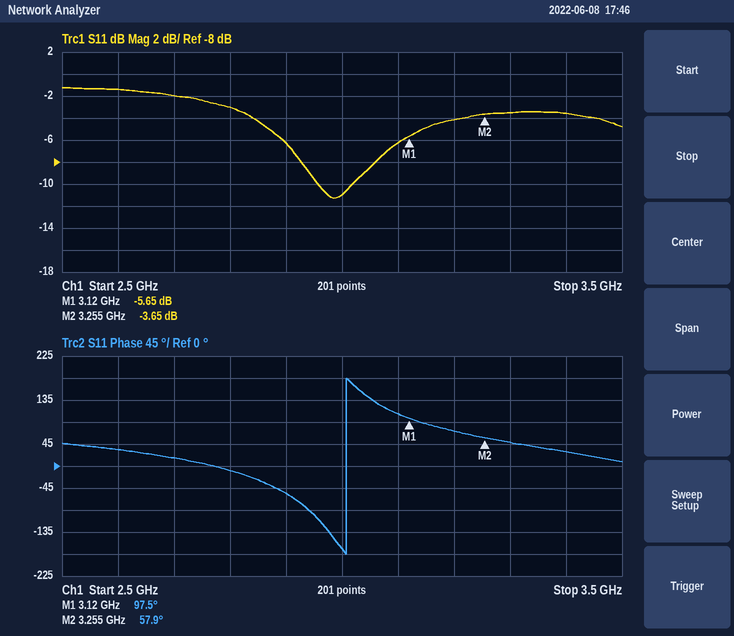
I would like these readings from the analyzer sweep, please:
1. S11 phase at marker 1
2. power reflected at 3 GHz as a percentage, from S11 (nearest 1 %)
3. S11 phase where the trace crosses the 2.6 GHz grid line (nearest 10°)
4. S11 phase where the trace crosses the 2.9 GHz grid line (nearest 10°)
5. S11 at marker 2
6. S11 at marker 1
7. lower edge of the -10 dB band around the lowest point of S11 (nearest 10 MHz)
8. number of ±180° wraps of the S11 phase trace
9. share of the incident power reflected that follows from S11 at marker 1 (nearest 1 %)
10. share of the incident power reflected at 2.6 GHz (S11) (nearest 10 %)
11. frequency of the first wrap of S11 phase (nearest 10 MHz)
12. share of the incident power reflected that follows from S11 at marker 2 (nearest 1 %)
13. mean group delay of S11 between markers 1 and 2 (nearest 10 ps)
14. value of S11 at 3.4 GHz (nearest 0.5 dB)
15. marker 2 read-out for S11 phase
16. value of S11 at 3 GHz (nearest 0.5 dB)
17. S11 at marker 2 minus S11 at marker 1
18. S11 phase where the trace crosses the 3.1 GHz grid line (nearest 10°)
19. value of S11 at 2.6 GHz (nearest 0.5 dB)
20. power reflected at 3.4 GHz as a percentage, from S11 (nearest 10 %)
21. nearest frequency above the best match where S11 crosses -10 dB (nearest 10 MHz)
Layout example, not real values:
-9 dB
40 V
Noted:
97.5°
8 %
30°
-60°
-3.65 dB
-5.65 dB
2.96 GHz
1
27 %
70 %
3.01 GHz
43 %
810 ps
-3.5 dB
57.9°
-11.0 dB
2.00 dB
110°
-1.5 dB
40 %
3.02 GHz
